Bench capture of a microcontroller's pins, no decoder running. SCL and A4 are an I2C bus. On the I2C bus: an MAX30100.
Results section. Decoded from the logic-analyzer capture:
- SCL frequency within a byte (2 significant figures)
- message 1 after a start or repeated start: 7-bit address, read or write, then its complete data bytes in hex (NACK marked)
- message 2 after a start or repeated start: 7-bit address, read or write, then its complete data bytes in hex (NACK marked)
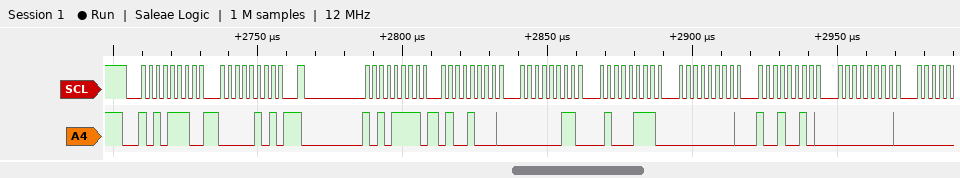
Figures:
400 kHz
0x57 write: 05
0x57 read: 48 03 47 00 92 00
